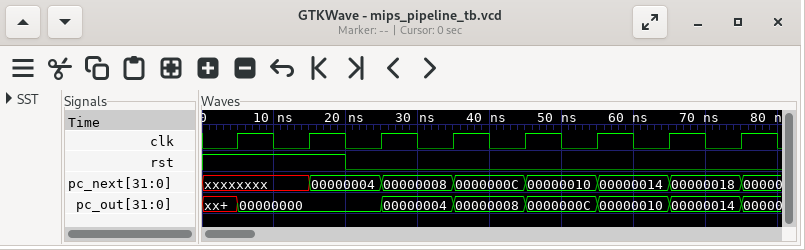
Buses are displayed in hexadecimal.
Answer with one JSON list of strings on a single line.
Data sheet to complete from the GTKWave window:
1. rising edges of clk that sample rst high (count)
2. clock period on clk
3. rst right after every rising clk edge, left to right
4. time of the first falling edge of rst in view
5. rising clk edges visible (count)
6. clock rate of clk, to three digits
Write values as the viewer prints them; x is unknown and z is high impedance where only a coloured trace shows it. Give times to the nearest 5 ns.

["2", "10 ns", "1 1 0 0 0 0 0 0", "20 ns", "8", "100 MHz"]
